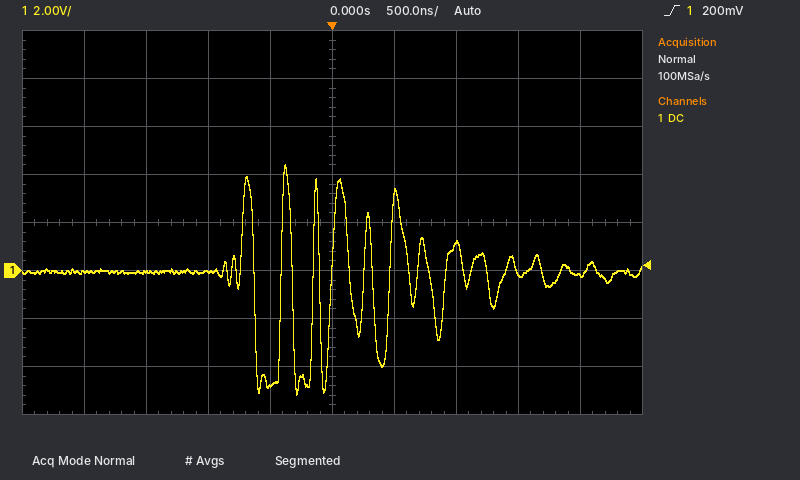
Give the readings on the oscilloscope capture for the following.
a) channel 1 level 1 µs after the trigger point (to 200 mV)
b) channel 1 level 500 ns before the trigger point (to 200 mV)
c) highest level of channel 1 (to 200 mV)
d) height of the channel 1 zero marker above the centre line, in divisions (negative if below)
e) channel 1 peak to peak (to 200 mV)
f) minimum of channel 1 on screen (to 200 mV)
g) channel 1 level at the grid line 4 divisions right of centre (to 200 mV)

1.0 V
-4.8 V
4.4 V
-1.0 div
9.6 V
-5.2 V
-200 mV
